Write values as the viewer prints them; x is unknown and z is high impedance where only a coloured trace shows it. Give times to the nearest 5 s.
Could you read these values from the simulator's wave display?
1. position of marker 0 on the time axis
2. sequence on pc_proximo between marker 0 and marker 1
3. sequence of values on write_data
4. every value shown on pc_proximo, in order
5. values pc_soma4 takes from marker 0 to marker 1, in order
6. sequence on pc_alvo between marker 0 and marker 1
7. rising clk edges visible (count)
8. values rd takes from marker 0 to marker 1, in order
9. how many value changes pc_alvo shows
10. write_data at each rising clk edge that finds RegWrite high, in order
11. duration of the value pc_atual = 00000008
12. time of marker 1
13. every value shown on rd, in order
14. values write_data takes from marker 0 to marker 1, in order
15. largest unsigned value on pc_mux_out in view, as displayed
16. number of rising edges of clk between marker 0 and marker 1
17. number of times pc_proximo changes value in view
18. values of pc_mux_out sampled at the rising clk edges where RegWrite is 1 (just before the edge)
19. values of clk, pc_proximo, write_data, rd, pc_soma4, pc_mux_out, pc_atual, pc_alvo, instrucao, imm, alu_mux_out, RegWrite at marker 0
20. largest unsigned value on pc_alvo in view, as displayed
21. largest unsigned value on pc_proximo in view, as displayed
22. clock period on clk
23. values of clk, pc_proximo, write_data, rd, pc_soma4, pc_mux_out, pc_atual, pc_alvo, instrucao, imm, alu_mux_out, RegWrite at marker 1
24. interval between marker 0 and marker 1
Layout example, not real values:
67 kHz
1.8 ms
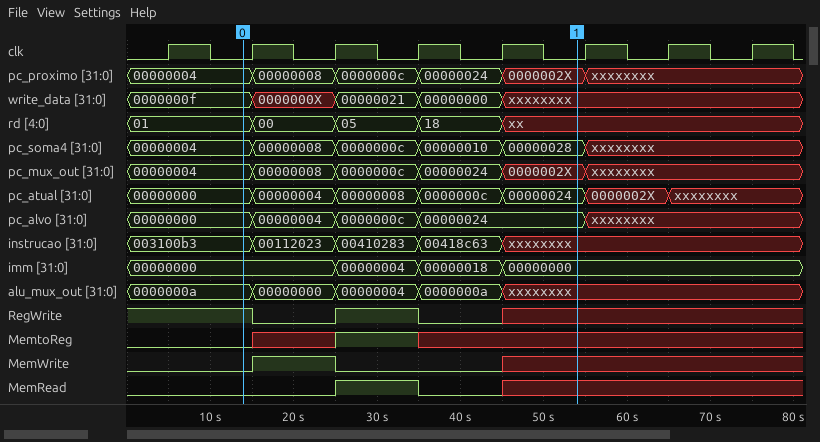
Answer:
15 s
00000004, 00000008, 0000000c, 00000024, 0000002X
0000000f, 0000000X, 00000021, 00000000, xxxxxxxx
00000004, 00000008, 0000000c, 00000024, 0000002X, xxxxxxxx
00000004, 00000008, 0000000c, 00000010, 00000028
00000000, 00000004, 0000000c, 00000024
8
01, 00, 05, 18, xx
4
0000000f, 0000000f, 00000021
10 s
55 s
01, 00, 05, 18, xx
0000000f, 0000000X, 00000021, 00000000, xxxxxxxx
00000024
4
5
00000004, 00000004, 0000000c
clk=0, pc_proximo=00000004, write_data=0000000f, rd=01, pc_soma4=00000004, pc_mux_out=00000004, pc_atual=00000000, pc_alvo=00000000, instrucao=003100b3, imm=00000000, alu_mux_out=0000000a, RegWrite=1
00000024
00000024
10 s
clk=0, pc_proximo=0000002X, write_data=xxxxxxxx, rd=xx, pc_soma4=00000028, pc_mux_out=0000002X, pc_atual=00000024, pc_alvo=00000024, instrucao=xxxxxxxx, imm=00000000, alu_mux_out=xxxxxxxx, RegWrite=x
40 s
